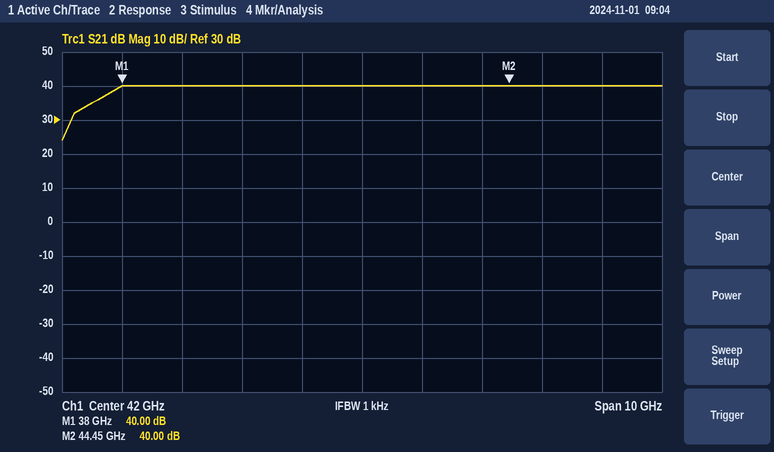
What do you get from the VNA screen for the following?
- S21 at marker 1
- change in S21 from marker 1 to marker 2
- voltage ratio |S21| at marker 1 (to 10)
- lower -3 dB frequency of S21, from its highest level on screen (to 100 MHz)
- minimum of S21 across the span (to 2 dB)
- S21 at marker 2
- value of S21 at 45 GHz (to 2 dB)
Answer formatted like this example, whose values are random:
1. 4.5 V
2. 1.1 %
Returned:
1. 40.00 dB
2. 0.00 dB
3. 100
4. 37.7 GHz
5. 24 dB
6. 40.00 dB
7. 40 dB
